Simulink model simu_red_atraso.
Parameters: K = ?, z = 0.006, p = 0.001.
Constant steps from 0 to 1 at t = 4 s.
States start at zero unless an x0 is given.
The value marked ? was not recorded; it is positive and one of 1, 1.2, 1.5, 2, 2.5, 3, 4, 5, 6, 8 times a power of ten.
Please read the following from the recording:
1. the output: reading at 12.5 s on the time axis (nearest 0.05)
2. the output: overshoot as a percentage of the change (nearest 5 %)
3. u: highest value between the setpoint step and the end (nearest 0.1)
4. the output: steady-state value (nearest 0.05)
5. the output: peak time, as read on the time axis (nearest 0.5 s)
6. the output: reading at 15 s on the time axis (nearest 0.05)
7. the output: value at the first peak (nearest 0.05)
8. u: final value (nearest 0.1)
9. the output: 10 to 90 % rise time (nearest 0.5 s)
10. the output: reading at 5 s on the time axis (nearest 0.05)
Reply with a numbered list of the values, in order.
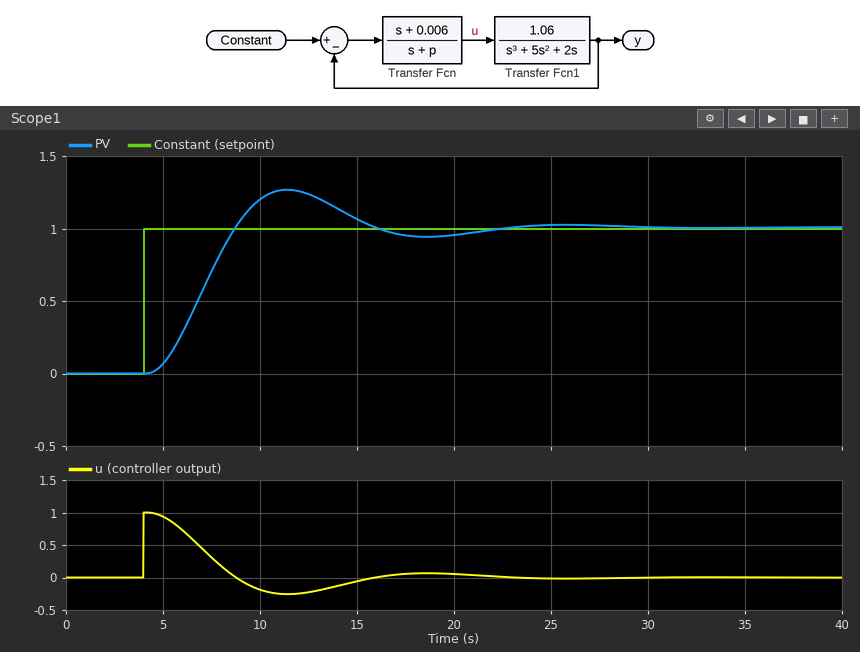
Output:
1. 1.25
2. 25 %
3. 1.0
4. 1.00
5. 11.5 s
6. 1.05
7. 1.25
8. 0.0
9. 3.0 s
10. 0.05
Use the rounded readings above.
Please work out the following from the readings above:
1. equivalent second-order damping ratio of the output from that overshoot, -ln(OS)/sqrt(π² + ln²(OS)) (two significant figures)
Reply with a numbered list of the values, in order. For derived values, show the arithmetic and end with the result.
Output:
1. ln(0.25) = -1.386; 1.386 / sqrt(9.870 + 1.922) = 0.40
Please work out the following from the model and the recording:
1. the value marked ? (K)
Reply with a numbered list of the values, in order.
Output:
1. 1
